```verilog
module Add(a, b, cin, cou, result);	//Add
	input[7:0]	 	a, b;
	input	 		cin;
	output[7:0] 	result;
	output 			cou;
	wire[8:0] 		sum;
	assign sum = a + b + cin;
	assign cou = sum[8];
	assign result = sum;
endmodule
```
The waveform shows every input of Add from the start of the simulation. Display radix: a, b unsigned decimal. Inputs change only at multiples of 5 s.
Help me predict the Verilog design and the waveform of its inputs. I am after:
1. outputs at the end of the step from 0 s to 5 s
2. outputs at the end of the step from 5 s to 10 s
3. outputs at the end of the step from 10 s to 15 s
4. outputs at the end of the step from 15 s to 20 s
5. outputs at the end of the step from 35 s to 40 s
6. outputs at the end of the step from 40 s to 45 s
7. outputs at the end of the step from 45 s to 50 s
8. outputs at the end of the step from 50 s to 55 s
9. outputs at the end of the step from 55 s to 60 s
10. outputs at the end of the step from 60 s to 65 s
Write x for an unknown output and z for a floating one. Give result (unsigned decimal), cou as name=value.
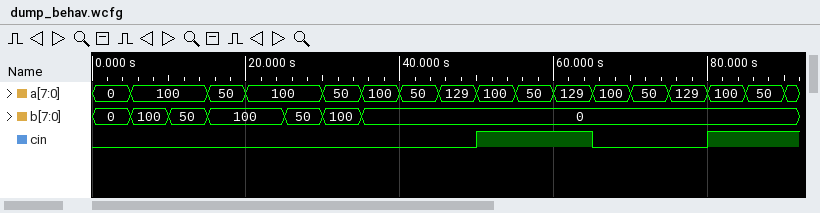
result=0, cou=0
result=200, cou=0
result=150, cou=0
result=150, cou=0
result=100, cou=0
result=50, cou=0
result=129, cou=0
result=101, cou=0
result=51, cou=0
result=130, cou=0
